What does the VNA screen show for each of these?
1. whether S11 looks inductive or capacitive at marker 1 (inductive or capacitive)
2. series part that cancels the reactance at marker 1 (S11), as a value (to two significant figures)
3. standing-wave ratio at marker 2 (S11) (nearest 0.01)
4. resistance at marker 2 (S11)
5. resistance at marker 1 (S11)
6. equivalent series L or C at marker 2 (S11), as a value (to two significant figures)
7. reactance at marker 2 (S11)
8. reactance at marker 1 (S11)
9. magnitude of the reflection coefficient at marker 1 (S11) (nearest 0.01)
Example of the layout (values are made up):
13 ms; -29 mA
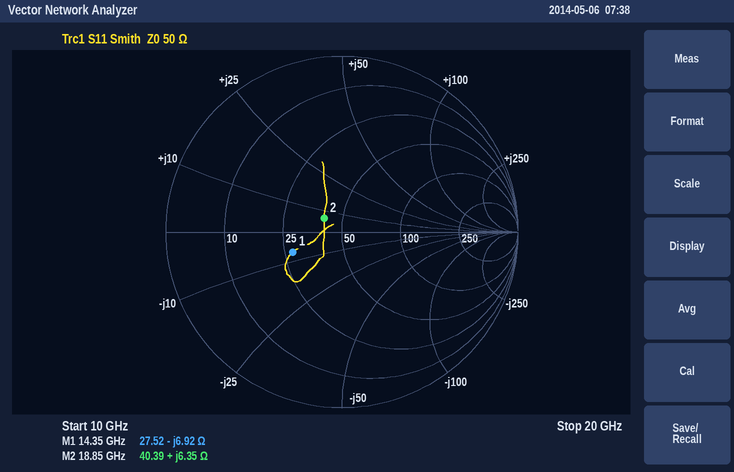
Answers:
capacitive; 77 pH; 1.29; 40.39 Ω; 27.52 Ω; 54 pH; +6.35 Ω; -6.92 Ω; 0.30
